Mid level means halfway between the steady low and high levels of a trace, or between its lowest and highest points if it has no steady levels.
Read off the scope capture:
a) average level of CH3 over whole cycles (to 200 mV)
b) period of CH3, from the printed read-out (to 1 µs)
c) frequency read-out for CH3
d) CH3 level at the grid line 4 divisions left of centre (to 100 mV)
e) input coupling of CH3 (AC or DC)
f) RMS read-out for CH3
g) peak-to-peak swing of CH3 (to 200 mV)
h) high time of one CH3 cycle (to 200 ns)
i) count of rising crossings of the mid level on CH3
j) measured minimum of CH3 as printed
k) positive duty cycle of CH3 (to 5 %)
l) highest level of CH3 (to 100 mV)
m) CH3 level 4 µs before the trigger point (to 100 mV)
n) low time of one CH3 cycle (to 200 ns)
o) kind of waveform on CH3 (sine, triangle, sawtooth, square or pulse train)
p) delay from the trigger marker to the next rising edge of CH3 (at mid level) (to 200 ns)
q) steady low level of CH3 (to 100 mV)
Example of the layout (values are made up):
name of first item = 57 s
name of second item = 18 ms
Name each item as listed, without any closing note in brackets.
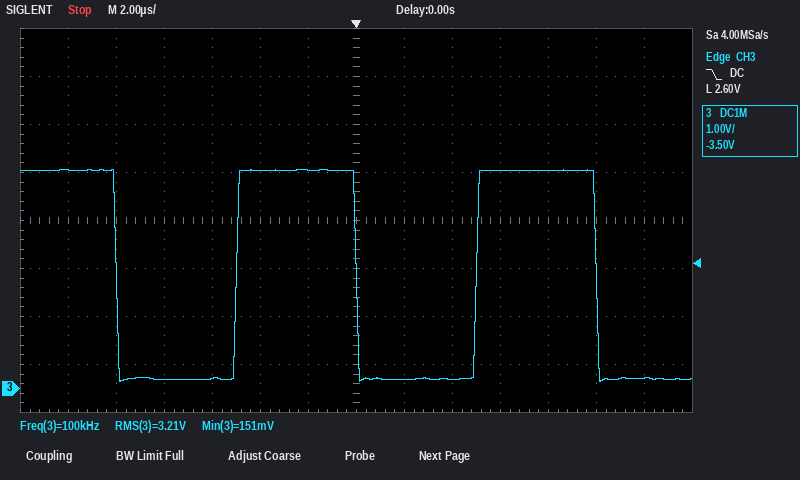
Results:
average level of CH3 over whole cycles = 2.4 V
period of CH3, from the printed read-out = 10 µs
frequency read-out for CH3 = 100 kHz
CH3 level at the grid line 4 divisions left of centre = 200 mV
input coupling of CH3 = DC
RMS read-out for CH3 = 3.21 V
peak-to-peak swing of CH3 = 4.4 V
high time of one CH3 cycle = 5.0 µs
count of rising crossings of the mid level on CH3 = 2
measured minimum of CH3 as printed = 151 mV
positive duty cycle of CH3 = 50 %
highest level of CH3 = 4.6 V
CH3 level 4 µs before the trigger point = 4.5 V
low time of one CH3 cycle = 5.0 µs
kind of waveform on CH3 = square
delay from the trigger marker to the next rising edge of CH3 (at mid level) = 5.0 µs
steady low level of CH3 = 200 mV
